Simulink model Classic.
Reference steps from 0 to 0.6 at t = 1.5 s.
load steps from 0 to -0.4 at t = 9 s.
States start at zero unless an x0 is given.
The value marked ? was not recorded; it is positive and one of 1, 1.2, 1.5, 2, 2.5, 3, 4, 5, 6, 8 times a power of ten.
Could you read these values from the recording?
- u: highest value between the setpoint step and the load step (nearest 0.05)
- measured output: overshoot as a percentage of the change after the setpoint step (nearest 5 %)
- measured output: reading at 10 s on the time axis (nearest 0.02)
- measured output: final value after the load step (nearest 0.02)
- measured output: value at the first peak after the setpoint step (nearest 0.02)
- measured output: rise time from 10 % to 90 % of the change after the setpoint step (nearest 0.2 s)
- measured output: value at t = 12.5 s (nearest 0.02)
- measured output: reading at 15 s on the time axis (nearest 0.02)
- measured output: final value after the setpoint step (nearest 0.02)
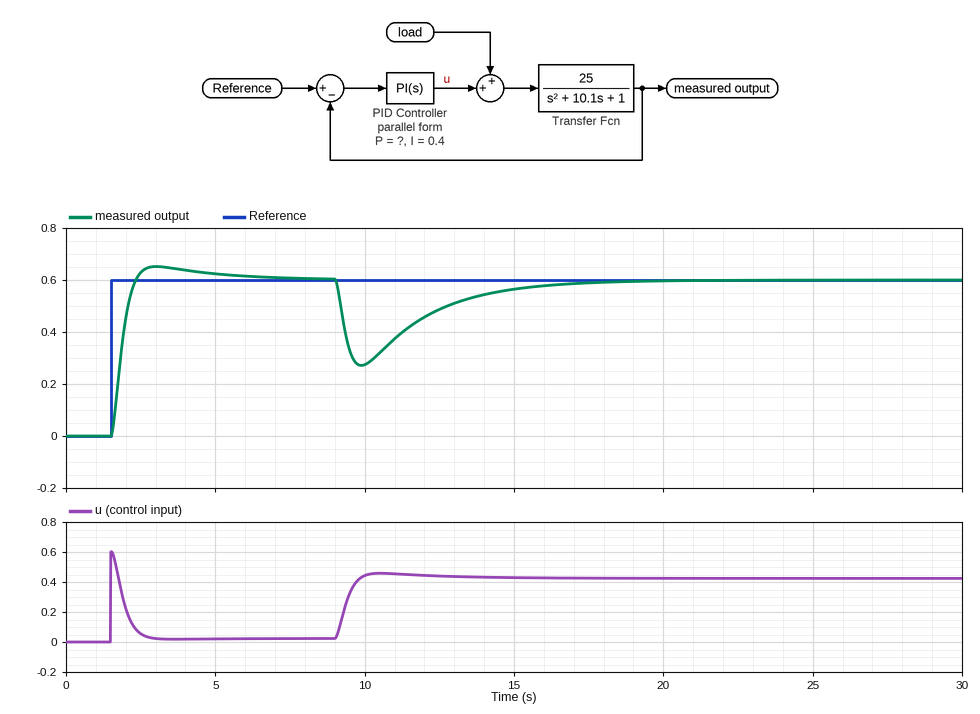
0.60
10 %
0.28
0.60
0.66
0.6 s
0.48
0.56
0.60
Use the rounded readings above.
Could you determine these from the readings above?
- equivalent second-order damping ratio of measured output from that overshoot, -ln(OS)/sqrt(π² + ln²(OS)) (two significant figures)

0.59
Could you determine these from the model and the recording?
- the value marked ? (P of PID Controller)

1
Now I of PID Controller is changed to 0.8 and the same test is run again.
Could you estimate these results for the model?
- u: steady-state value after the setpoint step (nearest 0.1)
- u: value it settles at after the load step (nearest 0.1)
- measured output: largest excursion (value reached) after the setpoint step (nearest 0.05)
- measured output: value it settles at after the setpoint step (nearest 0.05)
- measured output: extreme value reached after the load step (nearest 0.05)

0.0
0.4
0.70
0.60
0.30
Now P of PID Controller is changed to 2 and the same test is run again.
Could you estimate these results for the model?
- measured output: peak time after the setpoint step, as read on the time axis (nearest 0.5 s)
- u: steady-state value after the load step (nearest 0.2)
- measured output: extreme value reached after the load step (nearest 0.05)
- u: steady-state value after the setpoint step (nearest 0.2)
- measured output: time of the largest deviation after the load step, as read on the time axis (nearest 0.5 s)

2.0 s
0.4
0.40
0.0
9.5 s
